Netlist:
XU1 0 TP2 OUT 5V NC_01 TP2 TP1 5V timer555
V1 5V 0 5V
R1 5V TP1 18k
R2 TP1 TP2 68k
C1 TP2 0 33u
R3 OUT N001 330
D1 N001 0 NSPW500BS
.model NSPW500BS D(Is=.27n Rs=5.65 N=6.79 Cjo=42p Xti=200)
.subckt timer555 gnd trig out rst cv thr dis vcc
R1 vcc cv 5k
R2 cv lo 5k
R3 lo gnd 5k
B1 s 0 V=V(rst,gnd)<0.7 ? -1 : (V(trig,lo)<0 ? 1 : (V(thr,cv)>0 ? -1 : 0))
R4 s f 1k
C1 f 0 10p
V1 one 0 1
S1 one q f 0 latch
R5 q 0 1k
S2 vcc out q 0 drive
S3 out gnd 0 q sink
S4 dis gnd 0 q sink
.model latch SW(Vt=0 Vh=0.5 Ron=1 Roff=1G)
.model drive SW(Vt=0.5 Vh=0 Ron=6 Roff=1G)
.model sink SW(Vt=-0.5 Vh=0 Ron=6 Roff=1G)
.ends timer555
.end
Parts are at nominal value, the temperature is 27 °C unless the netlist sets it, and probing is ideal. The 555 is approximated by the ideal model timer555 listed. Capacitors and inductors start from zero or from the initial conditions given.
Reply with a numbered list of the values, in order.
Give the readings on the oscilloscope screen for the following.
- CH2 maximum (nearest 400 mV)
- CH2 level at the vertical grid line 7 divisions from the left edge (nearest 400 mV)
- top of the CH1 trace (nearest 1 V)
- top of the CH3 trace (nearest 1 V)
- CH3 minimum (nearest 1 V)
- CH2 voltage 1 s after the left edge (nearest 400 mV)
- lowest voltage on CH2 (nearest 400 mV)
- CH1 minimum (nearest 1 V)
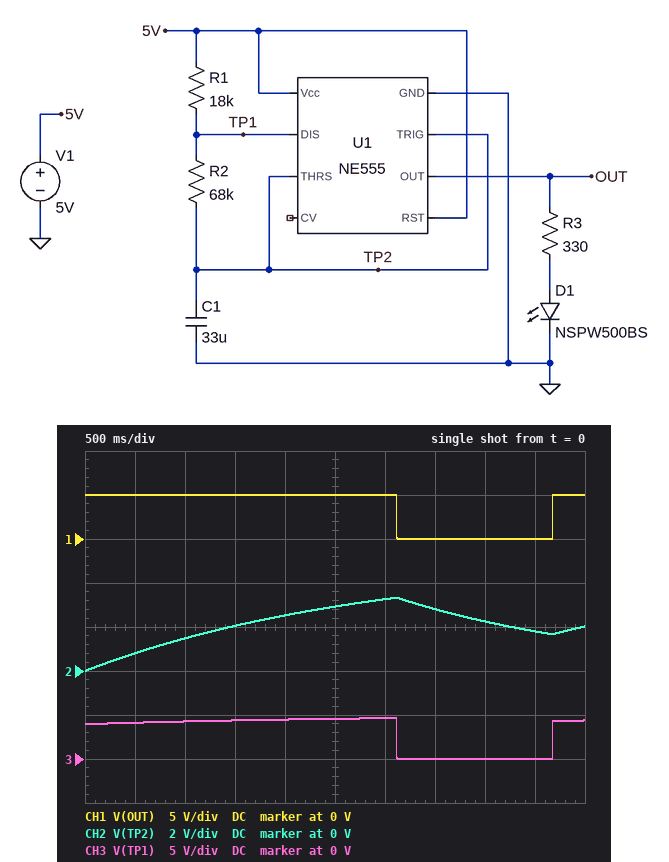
1. 3.2 V
2. 2.8 V
3. 5 V
4. 5 V
5. 0 V
6. 1.6 V
7. 0 V
8. 0 V
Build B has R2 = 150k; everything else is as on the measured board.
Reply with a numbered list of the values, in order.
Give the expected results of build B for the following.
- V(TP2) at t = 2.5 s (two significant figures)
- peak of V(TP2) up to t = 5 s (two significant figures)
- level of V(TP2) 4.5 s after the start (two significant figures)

1. 1.8 V
2. 3.0 V
3. 2.8 V
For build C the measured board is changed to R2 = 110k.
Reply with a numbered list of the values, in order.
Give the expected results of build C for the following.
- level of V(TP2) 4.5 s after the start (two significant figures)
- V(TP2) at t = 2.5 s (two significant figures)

1. 3.3 V
2. 2.2 V
